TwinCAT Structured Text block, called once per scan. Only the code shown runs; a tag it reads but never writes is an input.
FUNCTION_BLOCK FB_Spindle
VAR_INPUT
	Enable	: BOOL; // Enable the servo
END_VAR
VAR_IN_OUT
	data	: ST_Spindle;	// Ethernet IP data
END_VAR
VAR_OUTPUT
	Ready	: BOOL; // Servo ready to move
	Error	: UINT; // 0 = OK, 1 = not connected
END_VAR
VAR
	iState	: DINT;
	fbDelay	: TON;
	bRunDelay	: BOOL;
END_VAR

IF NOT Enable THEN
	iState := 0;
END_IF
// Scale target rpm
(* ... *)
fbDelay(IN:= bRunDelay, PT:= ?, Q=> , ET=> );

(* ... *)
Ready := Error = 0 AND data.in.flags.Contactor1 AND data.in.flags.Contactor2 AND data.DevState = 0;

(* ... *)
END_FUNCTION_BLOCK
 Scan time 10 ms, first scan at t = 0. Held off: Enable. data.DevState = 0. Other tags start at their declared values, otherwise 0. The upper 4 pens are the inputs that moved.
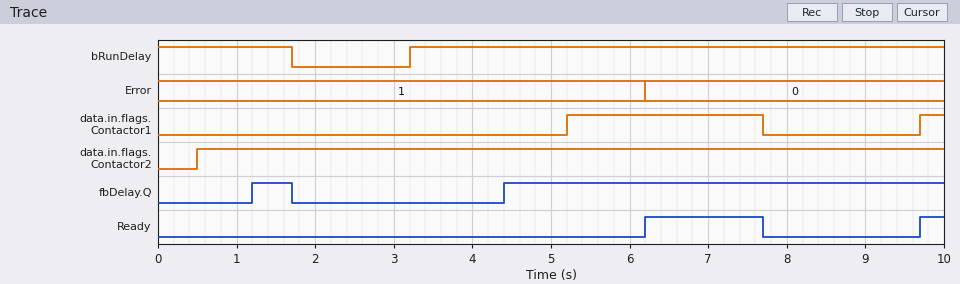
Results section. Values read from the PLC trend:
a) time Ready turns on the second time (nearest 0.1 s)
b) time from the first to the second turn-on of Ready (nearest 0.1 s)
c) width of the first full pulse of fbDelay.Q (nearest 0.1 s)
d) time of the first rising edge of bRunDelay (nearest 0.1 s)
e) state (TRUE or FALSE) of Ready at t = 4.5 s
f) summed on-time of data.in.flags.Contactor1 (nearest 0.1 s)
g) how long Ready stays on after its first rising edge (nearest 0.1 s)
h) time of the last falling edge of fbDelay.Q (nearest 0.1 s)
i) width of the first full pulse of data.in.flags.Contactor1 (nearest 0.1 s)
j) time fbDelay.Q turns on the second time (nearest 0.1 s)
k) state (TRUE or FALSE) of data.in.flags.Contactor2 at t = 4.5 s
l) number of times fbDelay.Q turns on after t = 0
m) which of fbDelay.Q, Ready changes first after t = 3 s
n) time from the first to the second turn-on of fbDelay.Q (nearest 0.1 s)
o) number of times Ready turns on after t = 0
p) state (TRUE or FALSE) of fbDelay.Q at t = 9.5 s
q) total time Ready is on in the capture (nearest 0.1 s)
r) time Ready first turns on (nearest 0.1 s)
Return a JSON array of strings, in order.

["9.7 s", "3.5 s", "0.5 s", "3.2 s", "FALSE", "2.8 s", "1.5 s", "1.7 s", "2.5 s", "4.4 s", "TRUE", "2", "fbDelay.Q", "3.2 s", "2", "TRUE", "1.8 s", "6.2 s"]
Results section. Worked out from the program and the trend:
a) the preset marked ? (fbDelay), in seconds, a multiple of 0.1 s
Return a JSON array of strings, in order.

["1.2 s"]
